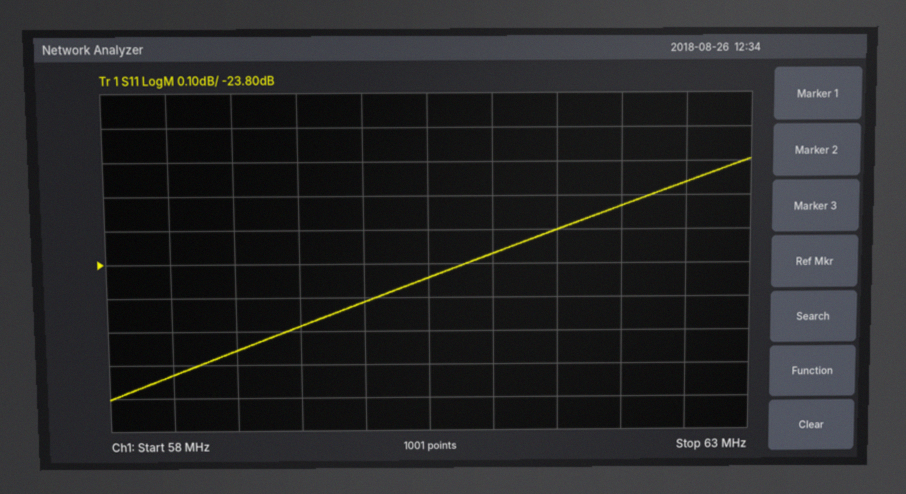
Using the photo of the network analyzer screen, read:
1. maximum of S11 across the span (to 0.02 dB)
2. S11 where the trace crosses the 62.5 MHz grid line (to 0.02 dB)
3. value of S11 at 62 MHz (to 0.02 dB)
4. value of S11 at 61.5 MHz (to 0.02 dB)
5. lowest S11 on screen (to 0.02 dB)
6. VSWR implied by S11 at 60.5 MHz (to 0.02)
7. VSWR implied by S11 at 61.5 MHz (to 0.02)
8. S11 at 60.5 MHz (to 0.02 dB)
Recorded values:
-23.50 dB
-23.56 dB
-23.64 dB
-23.70 dB
-24.20 dB
1.14
1.14
-23.84 dB
